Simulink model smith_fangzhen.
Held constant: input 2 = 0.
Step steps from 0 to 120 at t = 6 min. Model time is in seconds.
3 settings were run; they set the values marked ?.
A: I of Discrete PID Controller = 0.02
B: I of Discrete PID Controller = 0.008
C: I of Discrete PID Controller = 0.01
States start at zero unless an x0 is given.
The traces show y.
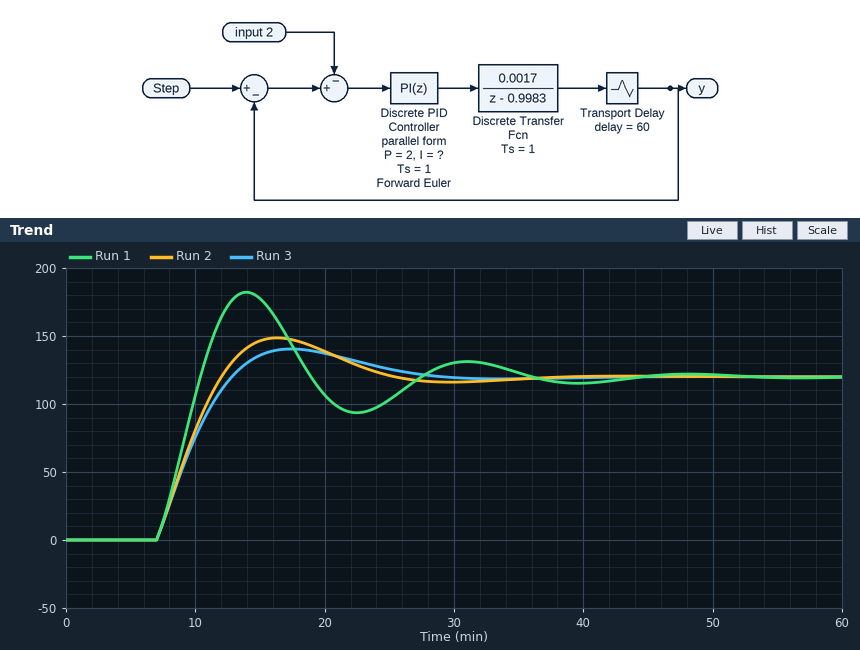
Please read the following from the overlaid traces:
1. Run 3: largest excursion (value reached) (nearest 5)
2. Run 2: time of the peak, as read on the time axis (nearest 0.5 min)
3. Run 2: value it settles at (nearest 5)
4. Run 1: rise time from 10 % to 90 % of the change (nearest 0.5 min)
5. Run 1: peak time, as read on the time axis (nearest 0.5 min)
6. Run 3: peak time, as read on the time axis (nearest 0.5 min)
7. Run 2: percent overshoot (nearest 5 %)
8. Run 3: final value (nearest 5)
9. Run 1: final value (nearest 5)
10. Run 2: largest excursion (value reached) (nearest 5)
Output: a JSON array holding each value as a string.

["140", "16.5 min", "120", "2.5 min", "14.0 min", "17.5 min", "25 %", "120", "120", "150"]
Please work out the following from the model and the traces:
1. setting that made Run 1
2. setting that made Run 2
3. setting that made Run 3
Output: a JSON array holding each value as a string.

["A", "C", "B"]
